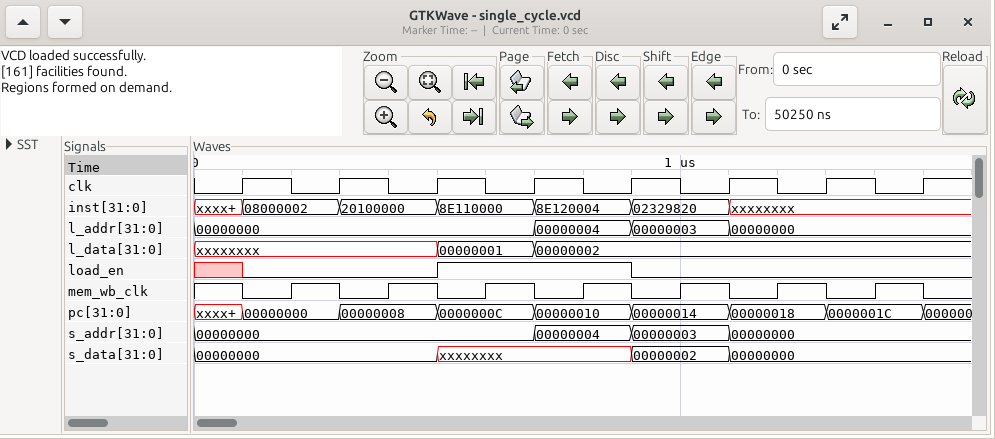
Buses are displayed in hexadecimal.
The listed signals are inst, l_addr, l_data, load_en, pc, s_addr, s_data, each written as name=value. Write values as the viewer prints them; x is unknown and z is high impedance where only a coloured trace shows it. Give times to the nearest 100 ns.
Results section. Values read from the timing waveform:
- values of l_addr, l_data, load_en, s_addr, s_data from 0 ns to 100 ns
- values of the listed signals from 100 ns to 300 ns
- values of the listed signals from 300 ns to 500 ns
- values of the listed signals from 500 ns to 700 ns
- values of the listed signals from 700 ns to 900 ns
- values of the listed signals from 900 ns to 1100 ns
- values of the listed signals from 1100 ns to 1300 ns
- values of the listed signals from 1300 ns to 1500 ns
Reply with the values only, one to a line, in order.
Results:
l_addr=00000000, l_data=xxxxxxxx, load_en=x, s_addr=00000000, s_data=00000000
inst=08000002, l_addr=00000000, l_data=xxxxxxxx, load_en=0, pc=00000000, s_addr=00000000, s_data=00000000
inst=20100000, l_addr=00000000, l_data=xxxxxxxx, load_en=0, pc=00000008, s_addr=00000000, s_data=00000000
inst=8E110000, l_addr=00000000, l_data=00000001, load_en=1, pc=0000000C, s_addr=00000000, s_data=xxxxxxxx
inst=8E120004, l_addr=00000004, l_data=00000002, load_en=1, pc=00000010, s_addr=00000004, s_data=xxxxxxxx
inst=02329820, l_addr=00000003, l_data=00000002, load_en=0, pc=00000014, s_addr=00000003, s_data=00000002
inst=xxxxxxxx, l_addr=00000000, l_data=00000002, load_en=0, pc=00000018, s_addr=00000000, s_data=00000000
inst=xxxxxxxx, l_addr=00000000, l_data=00000002, load_en=0, pc=0000001C, s_addr=00000000, s_data=00000000
